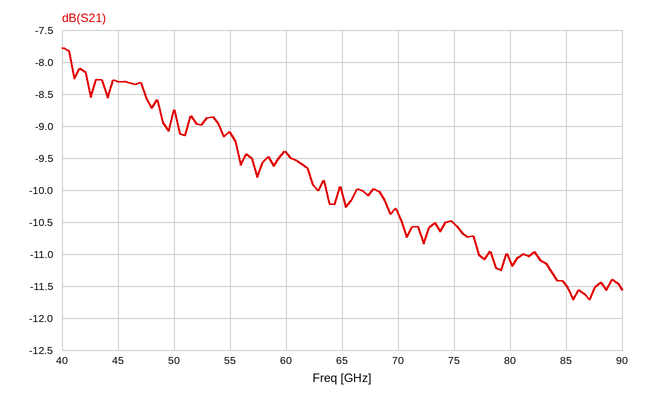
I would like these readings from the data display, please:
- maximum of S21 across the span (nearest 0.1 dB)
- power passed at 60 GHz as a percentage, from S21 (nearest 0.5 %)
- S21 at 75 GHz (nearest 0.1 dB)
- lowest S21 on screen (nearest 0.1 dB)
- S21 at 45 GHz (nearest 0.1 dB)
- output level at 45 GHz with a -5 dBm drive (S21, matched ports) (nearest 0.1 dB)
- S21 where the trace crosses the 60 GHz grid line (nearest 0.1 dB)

-7.8 dB
11.5 %
-10.5 dB
-11.7 dB
-8.3 dB
-13.3 dBm
-9.4 dB
